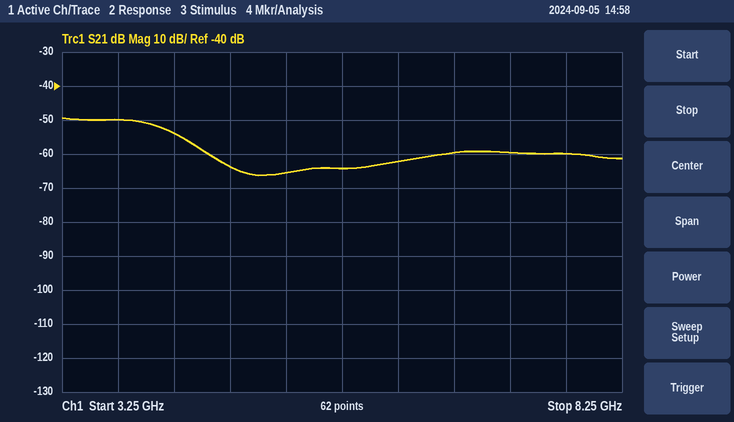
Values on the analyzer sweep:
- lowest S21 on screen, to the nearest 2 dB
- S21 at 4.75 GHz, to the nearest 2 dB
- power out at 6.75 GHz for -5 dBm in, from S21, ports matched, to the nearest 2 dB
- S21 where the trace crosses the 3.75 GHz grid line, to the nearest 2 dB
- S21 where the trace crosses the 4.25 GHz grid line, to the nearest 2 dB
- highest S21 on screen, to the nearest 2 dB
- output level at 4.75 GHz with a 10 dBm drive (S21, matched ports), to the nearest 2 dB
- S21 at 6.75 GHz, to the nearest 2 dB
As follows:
-66 dB
-64 dB
-64 dBm
-50 dB
-54 dB
-50 dB
-54 dBm
-60 dB
